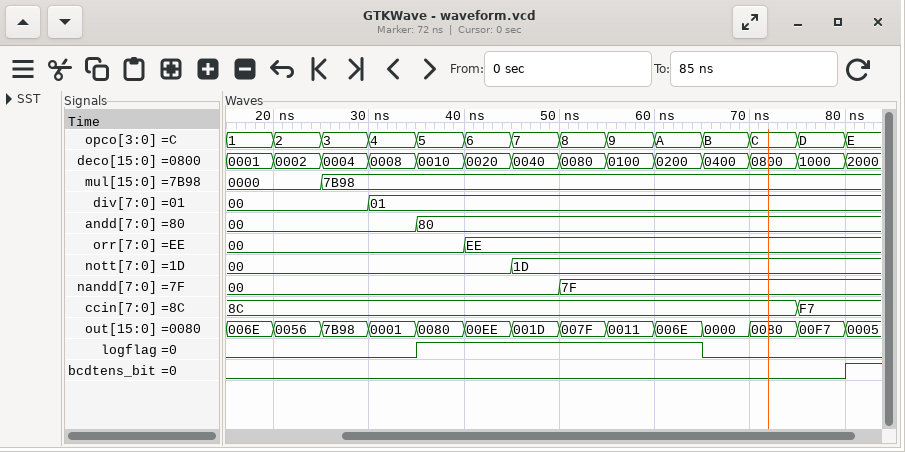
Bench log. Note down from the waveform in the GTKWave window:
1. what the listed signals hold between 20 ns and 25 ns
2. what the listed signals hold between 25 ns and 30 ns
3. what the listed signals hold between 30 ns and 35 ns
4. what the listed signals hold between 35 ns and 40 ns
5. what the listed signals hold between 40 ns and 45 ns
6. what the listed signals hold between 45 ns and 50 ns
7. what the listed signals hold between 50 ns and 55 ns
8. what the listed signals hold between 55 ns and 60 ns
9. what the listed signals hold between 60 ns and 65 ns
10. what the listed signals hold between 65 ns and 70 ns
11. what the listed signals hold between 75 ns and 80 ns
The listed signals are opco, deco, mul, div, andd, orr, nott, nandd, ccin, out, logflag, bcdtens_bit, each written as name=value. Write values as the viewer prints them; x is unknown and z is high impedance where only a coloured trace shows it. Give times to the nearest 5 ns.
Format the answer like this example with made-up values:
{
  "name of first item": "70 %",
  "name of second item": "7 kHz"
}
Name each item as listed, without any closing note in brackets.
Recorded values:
{
  "what the listed signals hold between 20 ns and 25 ns": "opco=2, deco=0002, mul=0000, div=00, andd=00, orr=00, nott=00, nandd=00, ccin=8C, out=0056, logflag=0, bcdtens_bit=0",
  "what the listed signals hold between 25 ns and 30 ns": "opco=3, deco=0004, mul=7B98, div=00, andd=00, orr=00, nott=00, nandd=00, ccin=8C, out=7B98, logflag=0, bcdtens_bit=0",
  "what the listed signals hold between 30 ns and 35 ns": "opco=4, deco=0008, mul=7B98, div=01, andd=00, orr=00, nott=00, nandd=00, ccin=8C, out=0001, logflag=0, bcdtens_bit=0",
  "what the listed signals hold between 35 ns and 40 ns": "opco=5, deco=0010, mul=7B98, div=01, andd=80, orr=00, nott=00, nandd=00, ccin=8C, out=0080, logflag=1, bcdtens_bit=0",
  "what the listed signals hold between 40 ns and 45 ns": "opco=6, deco=0020, mul=7B98, div=01, andd=80, orr=EE, nott=00, nandd=00, ccin=8C, out=00EE, logflag=1, bcdtens_bit=0",
  "what the listed signals hold between 45 ns and 50 ns": "opco=7, deco=0040, mul=7B98, div=01, andd=80, orr=EE, nott=1D, nandd=00, ccin=8C, out=001D, logflag=1, bcdtens_bit=0",
  "what the listed signals hold between 50 ns and 55 ns": "opco=8, deco=0080, mul=7B98, div=01, andd=80, orr=EE, nott=1D, nandd=7F, ccin=8C, out=007F, logflag=1, bcdtens_bit=0",
  "what the listed signals hold between 55 ns and 60 ns": "opco=9, deco=0100, mul=7B98, div=01, andd=80, orr=EE, nott=1D, nandd=7F, ccin=8C, out=0011, logflag=1, bcdtens_bit=0",
  "what the listed signals hold between 60 ns and 65 ns": "opco=A, deco=0200, mul=7B98, div=01, andd=80, orr=EE, nott=1D, nandd=7F, ccin=8C, out=006E, logflag=1, bcdtens_bit=0",
  "what the listed signals hold between 65 ns and 70 ns": "opco=B, deco=0400, mul=7B98, div=01, andd=80, orr=EE, nott=1D, nandd=7F, ccin=8C, out=0000, logflag=0, bcdtens_bit=0",
  "what the listed signals hold between 75 ns and 80 ns": "opco=D, deco=1000, mul=7B98, div=01, andd=80, orr=EE, nott=1D, nandd=7F, ccin=F7, out=00F7, logflag=0, bcdtens_bit=0"
}
